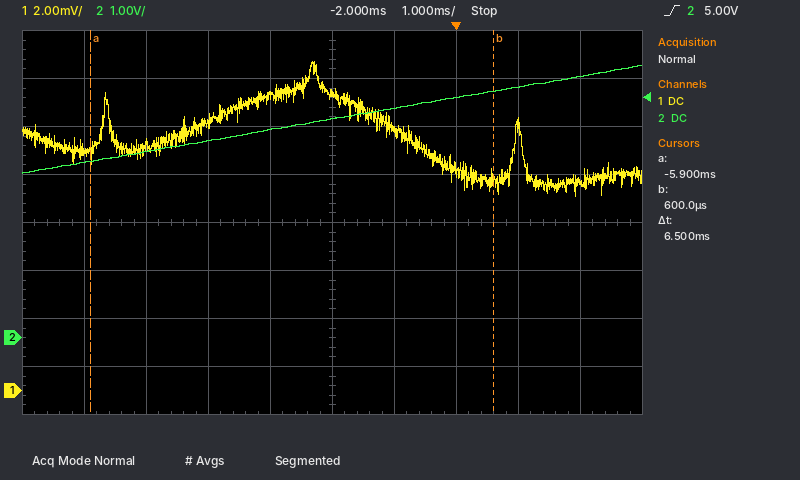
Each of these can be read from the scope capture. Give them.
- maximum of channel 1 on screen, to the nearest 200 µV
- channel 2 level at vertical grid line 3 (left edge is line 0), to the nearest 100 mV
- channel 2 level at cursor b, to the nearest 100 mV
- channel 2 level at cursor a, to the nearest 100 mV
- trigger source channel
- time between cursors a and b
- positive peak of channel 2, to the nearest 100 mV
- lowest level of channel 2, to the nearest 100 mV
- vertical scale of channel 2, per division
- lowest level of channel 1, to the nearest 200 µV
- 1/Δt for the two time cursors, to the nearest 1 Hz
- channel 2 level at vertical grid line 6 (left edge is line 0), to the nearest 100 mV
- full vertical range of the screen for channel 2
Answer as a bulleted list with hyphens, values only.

- 13.8 mV
- 4.1 V
- 5.1 V
- 3.7 V
- channel 2
- 6.5 ms
- 5.7 V
- 3.4 V
- 1 V
- 8.0 mV
- 154 Hz
- 4.8 V
- 8 V
